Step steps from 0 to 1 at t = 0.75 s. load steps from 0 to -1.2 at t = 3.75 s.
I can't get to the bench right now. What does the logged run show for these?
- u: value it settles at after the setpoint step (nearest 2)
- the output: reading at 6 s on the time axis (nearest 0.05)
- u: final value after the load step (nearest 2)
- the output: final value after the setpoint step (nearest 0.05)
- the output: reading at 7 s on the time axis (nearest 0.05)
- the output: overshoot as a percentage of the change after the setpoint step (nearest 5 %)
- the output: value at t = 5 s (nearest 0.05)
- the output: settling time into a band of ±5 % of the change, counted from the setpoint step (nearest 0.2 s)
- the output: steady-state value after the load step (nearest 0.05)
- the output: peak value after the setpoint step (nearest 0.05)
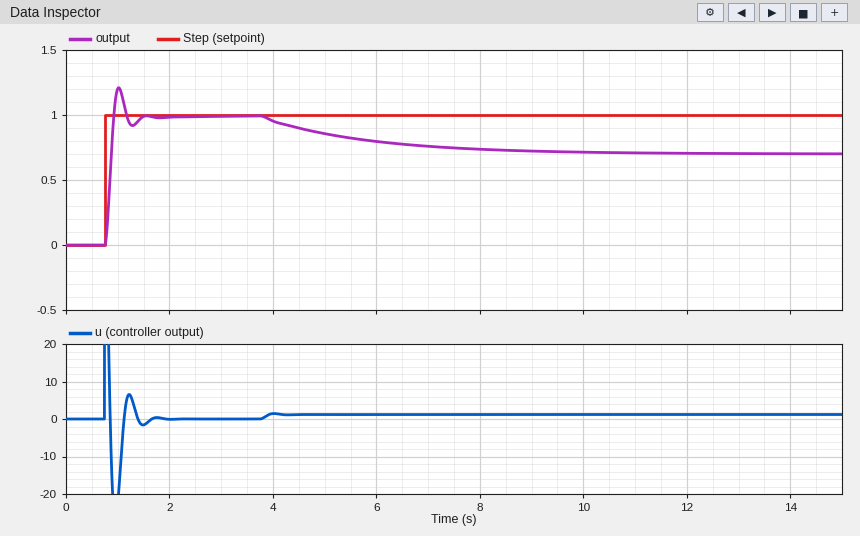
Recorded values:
0
0.80
2
1.00
0.75
20 %
0.85
0.6 s
0.70
1.20
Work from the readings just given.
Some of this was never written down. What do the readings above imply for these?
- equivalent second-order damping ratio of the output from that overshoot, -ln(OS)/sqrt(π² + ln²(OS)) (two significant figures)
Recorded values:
0.46
